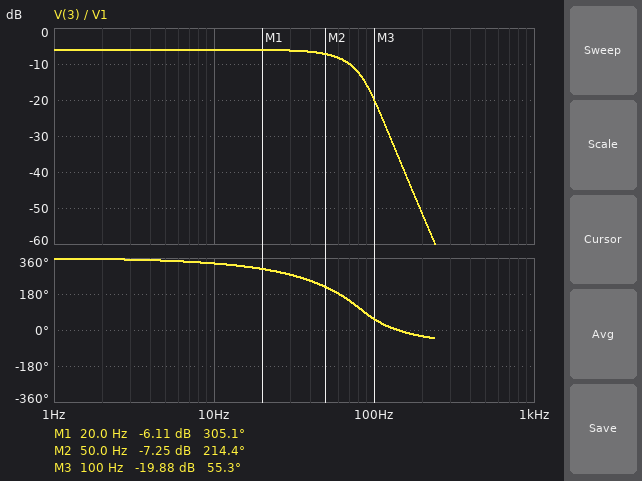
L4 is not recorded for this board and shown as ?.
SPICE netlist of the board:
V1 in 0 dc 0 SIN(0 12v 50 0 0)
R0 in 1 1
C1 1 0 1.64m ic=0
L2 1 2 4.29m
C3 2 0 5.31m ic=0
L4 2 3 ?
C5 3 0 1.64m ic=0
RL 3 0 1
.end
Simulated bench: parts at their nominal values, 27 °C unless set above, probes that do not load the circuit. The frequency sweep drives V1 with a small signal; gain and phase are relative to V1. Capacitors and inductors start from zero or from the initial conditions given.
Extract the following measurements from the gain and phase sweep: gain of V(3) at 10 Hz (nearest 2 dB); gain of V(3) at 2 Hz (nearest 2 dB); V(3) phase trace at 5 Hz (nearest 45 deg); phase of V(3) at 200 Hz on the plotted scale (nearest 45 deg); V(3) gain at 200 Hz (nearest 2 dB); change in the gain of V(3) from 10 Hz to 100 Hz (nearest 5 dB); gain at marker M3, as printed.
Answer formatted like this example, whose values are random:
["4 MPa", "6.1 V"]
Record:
["-6 dB", "-6 dB", "360 deg", "-45 deg", "-52 dB", "-15 dB", "-19.88 dB"]
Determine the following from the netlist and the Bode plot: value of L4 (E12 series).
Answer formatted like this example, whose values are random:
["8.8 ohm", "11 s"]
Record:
["2.2 mH"]
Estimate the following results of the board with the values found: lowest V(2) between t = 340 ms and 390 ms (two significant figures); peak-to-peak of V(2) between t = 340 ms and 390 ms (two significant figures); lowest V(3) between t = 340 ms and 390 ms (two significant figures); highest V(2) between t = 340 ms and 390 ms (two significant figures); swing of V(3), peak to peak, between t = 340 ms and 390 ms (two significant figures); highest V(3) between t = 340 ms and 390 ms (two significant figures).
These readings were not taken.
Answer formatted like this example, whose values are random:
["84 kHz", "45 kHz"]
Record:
["-4.9 V", "9.8 V", "-5.2 V", "4.9 V", "10 V", "5.2 V"]
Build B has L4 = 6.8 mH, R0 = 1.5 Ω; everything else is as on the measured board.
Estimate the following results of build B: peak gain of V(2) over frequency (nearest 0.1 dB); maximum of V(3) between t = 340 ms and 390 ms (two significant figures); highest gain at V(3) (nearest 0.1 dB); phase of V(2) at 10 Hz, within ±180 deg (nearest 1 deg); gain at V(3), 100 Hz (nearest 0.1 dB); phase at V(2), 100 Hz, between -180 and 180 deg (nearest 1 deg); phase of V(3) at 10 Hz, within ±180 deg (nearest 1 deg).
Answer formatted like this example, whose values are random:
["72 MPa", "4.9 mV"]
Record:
["-4.5 dB", "3.3 V", "-7.8 dB", "-11 deg", "-34.6 dB", "138 deg", "-35 deg"]
